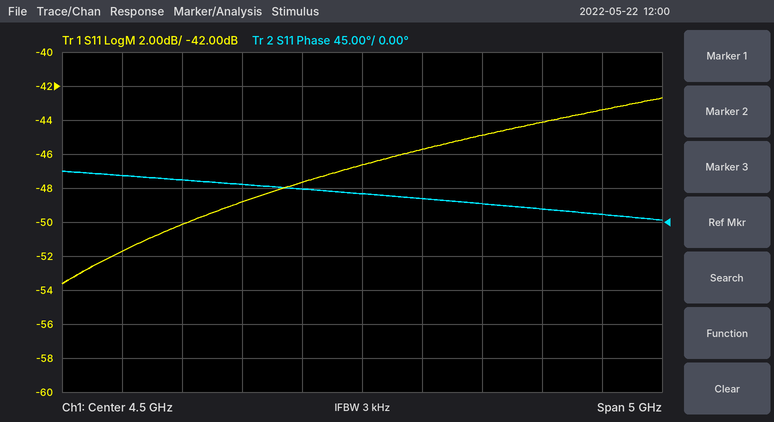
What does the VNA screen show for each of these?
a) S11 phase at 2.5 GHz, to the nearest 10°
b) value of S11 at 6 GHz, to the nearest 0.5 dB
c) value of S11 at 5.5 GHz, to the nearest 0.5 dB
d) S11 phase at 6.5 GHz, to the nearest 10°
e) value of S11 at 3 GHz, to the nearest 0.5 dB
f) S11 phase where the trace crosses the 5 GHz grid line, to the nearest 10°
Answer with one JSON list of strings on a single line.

["60°", "-44.0 dB", "-45.0 dB", "10°", "-50.0 dB", "30°"]
